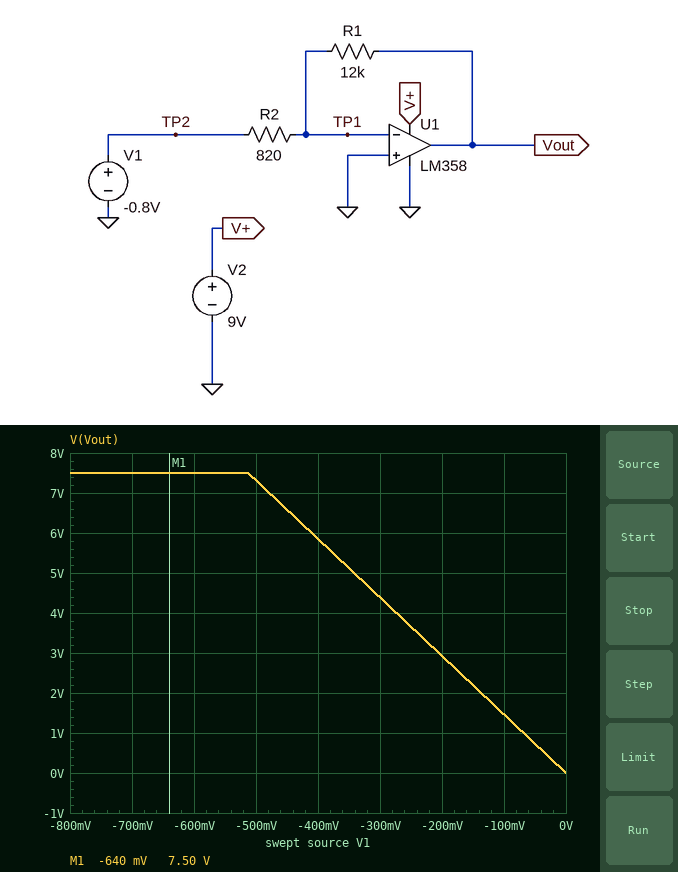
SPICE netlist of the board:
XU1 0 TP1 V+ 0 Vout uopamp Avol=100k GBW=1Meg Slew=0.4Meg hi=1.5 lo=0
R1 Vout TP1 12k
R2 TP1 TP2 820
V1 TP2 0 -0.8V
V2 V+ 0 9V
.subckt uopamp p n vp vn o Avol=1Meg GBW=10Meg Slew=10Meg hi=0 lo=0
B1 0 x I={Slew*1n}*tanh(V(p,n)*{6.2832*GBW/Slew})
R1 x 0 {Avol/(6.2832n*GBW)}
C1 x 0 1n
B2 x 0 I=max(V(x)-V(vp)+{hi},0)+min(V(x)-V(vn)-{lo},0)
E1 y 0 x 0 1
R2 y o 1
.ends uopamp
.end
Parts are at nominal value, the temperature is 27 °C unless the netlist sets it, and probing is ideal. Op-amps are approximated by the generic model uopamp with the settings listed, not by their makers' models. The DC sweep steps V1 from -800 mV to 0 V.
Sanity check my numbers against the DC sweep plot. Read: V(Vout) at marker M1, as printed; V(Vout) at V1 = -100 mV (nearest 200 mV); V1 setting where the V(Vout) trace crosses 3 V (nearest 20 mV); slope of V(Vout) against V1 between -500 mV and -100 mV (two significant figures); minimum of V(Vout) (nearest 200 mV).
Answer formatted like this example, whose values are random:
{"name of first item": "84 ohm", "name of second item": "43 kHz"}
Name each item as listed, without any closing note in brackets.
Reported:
{"V(Vout) at marker M1, as printed": "7.50 V", "V(Vout) at V1 = -100 mV": "1.4 V", "V1 setting where the V(Vout) trace crosses 3 V": "-200 mV", "slope of V(Vout) against V1 between -500 mV and -100 mV": "-15 V/V", "minimum of V(Vout)": "0 V"}
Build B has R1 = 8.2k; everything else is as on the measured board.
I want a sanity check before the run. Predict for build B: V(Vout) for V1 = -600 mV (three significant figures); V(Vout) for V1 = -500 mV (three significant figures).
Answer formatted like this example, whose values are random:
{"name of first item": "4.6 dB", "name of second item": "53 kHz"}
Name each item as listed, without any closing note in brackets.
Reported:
{"V(Vout) for V1 = -600 mV": "6.00 V", "V(Vout) for V1 = -500 mV": "5.00 V"}
